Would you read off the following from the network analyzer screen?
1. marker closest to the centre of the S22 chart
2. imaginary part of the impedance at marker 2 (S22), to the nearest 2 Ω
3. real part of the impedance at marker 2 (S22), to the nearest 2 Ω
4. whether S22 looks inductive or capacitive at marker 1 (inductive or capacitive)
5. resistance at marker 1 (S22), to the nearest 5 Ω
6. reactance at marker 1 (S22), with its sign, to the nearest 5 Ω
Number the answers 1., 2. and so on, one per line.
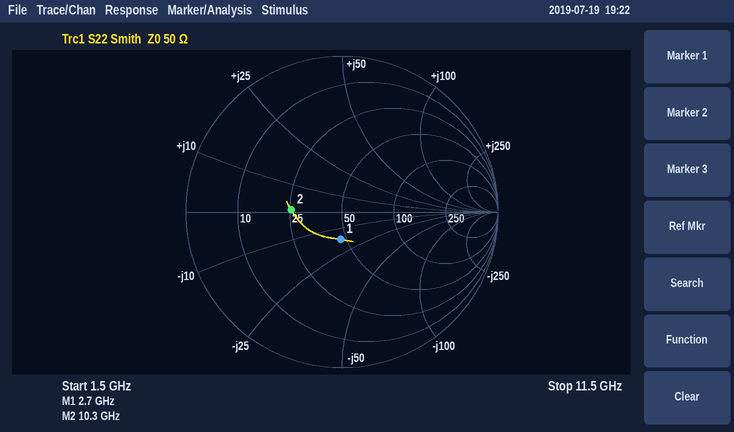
1. marker 1
2. 0 Ω
3. 26 Ω
4. capacitive
5. 45 Ω
6. -15 Ω
